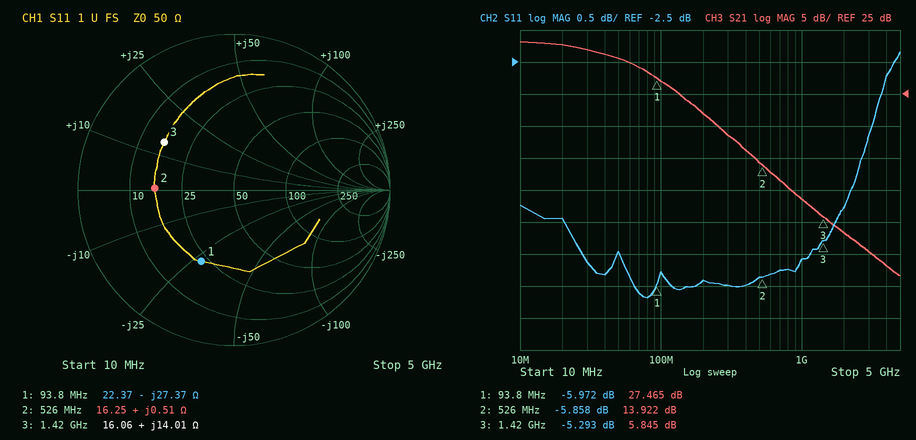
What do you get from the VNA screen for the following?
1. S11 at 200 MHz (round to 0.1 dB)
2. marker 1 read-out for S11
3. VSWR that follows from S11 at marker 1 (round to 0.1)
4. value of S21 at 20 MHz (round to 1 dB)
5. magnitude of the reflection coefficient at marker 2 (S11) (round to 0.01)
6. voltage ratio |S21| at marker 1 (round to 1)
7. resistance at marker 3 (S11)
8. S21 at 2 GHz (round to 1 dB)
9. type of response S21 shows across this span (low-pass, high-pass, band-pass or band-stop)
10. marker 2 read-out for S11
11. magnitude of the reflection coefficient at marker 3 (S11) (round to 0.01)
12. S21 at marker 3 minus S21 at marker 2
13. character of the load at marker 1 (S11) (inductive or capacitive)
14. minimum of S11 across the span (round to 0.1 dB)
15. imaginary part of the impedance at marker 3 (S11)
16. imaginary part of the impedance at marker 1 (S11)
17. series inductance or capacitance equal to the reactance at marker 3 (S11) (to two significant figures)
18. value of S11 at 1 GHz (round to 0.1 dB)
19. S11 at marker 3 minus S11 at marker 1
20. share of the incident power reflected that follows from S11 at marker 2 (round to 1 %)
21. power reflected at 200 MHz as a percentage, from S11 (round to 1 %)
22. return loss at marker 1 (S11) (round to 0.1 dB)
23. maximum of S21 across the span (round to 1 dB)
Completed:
-5.9 dB
-5.972 dB
3.0
33 dB
0.51
24
16.06 Ω
3 dB
low-pass
-5.858 dB
0.54
-8.077 dB
capacitive
-6.2 dB
+14.01 Ω
-27.37 Ω
1.6 nH
-5.6 dB
0.679 dB
26 %
26 %
6.0 dB
33 dB
